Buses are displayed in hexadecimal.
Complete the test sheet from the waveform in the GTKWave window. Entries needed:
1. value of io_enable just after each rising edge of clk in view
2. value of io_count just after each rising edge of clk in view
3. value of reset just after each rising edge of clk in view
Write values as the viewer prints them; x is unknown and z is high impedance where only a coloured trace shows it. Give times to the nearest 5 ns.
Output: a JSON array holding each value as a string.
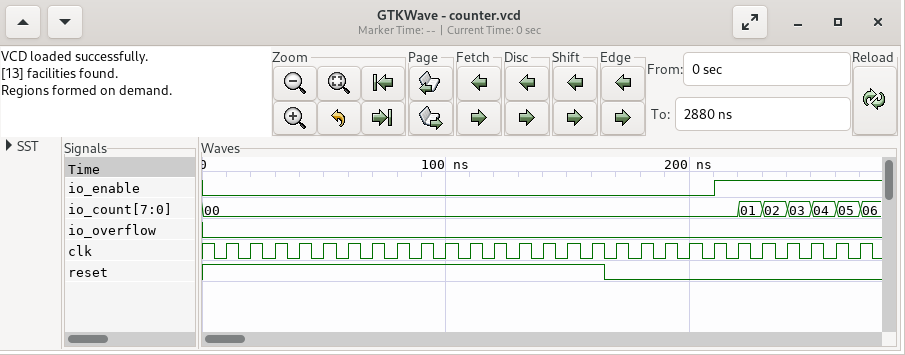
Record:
["0 0 0 0 0 0 0 0 0 0 0 0 0 0 0 0 0 0 0 0 1 1 1 1 1 1 1", "00, 00, 00, 00, 00, 00, 00, 00, 00, 00, 00, 00, 00, 00, 00, 00, 00, 00, 00, 00, 00, 01, 02, 03, 04, 05, 06", "1 1 1 1 1 1 1 1 1 1 1 1 1 1 1 1 0 0 0 0 0 0 0 0 0 0 0"]
